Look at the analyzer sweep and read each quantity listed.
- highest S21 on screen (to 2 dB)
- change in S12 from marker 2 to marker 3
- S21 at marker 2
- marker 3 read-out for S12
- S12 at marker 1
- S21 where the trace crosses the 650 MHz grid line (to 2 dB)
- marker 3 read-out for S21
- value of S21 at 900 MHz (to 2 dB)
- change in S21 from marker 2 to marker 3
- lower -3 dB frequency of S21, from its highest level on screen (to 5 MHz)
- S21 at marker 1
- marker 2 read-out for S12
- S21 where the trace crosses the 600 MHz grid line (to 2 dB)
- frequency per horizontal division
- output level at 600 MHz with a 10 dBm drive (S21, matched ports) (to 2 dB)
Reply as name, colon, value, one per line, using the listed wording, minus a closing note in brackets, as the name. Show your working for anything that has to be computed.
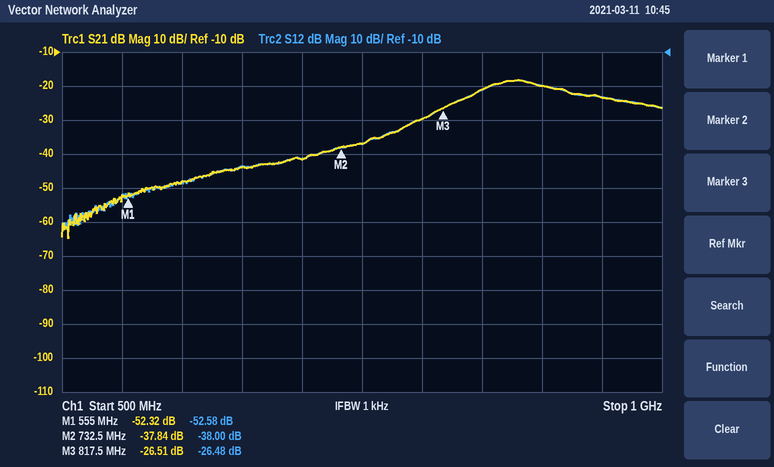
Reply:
highest S21 on screen: -18 dB
change in S12 from marker 2 to marker 3: -26.48 − (-38) = 11.52 dB
S21 at marker 2: -37.84 dB
marker 3 read-out for S12: -26.48 dB
S12 at marker 1: -52.58 dB
S21 where the trace crosses the 650 MHz grid line: -44 dB
marker 3 read-out for S21: -26.51 dB
value of S21 at 900 MHz: -20 dB
change in S21 from marker 2 to marker 3: -26.51 − (-37.84) = 11.33 dB
lower -3 dB frequency of S21, from its highest level on screen: 850 MHz
S21 at marker 1: -52.32 dB
marker 2 read-out for S12: -38.00 dB
S21 where the trace crosses the 600 MHz grid line: -48 dB
frequency per horizontal division: 50 MHz
output level at 600 MHz with a 10 dBm drive (S21, matched ports): 10 dBm + (-48 dB) = -38 dBm
